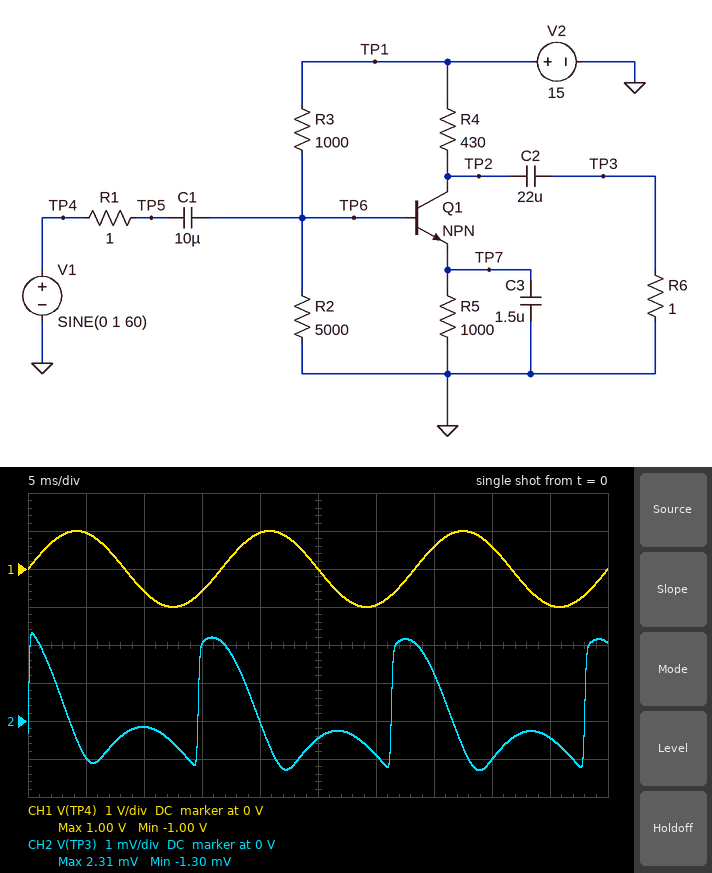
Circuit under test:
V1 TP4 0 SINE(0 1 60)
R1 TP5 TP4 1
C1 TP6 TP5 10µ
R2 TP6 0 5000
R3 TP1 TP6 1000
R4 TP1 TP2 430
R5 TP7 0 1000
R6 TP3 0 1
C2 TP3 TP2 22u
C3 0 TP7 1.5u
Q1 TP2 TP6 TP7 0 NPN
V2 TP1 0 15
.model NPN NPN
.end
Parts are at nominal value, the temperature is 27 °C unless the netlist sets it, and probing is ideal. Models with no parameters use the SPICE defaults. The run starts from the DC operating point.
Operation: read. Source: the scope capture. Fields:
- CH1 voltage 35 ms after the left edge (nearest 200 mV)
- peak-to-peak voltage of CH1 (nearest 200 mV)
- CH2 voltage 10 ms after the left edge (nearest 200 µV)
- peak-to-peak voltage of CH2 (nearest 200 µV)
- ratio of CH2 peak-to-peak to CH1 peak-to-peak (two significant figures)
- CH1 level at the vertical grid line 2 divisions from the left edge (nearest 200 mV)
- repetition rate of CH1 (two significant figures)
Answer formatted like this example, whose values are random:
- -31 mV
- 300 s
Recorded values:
- 600 mV
- 2.0 V
- -200 µV
- 3.6 mV
- 0.0018
- -600 mV
- 60 Hz
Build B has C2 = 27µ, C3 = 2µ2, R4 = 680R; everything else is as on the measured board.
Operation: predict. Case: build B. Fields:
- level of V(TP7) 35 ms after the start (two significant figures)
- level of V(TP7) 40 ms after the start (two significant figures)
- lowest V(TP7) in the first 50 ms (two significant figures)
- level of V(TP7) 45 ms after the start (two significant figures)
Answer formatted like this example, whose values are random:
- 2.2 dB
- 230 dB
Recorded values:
- 10 V
- 9.9 V
- 9.4 V
- 9.5 V
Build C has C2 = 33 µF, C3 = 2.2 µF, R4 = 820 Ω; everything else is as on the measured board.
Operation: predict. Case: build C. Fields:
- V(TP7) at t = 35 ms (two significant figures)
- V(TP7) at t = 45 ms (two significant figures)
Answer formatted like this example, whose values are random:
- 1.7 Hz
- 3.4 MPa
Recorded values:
- 9.6 V
- 9.2 V
